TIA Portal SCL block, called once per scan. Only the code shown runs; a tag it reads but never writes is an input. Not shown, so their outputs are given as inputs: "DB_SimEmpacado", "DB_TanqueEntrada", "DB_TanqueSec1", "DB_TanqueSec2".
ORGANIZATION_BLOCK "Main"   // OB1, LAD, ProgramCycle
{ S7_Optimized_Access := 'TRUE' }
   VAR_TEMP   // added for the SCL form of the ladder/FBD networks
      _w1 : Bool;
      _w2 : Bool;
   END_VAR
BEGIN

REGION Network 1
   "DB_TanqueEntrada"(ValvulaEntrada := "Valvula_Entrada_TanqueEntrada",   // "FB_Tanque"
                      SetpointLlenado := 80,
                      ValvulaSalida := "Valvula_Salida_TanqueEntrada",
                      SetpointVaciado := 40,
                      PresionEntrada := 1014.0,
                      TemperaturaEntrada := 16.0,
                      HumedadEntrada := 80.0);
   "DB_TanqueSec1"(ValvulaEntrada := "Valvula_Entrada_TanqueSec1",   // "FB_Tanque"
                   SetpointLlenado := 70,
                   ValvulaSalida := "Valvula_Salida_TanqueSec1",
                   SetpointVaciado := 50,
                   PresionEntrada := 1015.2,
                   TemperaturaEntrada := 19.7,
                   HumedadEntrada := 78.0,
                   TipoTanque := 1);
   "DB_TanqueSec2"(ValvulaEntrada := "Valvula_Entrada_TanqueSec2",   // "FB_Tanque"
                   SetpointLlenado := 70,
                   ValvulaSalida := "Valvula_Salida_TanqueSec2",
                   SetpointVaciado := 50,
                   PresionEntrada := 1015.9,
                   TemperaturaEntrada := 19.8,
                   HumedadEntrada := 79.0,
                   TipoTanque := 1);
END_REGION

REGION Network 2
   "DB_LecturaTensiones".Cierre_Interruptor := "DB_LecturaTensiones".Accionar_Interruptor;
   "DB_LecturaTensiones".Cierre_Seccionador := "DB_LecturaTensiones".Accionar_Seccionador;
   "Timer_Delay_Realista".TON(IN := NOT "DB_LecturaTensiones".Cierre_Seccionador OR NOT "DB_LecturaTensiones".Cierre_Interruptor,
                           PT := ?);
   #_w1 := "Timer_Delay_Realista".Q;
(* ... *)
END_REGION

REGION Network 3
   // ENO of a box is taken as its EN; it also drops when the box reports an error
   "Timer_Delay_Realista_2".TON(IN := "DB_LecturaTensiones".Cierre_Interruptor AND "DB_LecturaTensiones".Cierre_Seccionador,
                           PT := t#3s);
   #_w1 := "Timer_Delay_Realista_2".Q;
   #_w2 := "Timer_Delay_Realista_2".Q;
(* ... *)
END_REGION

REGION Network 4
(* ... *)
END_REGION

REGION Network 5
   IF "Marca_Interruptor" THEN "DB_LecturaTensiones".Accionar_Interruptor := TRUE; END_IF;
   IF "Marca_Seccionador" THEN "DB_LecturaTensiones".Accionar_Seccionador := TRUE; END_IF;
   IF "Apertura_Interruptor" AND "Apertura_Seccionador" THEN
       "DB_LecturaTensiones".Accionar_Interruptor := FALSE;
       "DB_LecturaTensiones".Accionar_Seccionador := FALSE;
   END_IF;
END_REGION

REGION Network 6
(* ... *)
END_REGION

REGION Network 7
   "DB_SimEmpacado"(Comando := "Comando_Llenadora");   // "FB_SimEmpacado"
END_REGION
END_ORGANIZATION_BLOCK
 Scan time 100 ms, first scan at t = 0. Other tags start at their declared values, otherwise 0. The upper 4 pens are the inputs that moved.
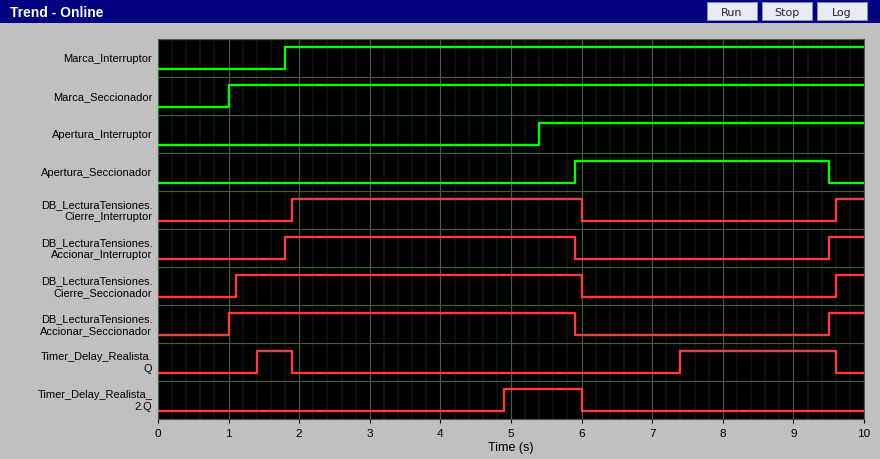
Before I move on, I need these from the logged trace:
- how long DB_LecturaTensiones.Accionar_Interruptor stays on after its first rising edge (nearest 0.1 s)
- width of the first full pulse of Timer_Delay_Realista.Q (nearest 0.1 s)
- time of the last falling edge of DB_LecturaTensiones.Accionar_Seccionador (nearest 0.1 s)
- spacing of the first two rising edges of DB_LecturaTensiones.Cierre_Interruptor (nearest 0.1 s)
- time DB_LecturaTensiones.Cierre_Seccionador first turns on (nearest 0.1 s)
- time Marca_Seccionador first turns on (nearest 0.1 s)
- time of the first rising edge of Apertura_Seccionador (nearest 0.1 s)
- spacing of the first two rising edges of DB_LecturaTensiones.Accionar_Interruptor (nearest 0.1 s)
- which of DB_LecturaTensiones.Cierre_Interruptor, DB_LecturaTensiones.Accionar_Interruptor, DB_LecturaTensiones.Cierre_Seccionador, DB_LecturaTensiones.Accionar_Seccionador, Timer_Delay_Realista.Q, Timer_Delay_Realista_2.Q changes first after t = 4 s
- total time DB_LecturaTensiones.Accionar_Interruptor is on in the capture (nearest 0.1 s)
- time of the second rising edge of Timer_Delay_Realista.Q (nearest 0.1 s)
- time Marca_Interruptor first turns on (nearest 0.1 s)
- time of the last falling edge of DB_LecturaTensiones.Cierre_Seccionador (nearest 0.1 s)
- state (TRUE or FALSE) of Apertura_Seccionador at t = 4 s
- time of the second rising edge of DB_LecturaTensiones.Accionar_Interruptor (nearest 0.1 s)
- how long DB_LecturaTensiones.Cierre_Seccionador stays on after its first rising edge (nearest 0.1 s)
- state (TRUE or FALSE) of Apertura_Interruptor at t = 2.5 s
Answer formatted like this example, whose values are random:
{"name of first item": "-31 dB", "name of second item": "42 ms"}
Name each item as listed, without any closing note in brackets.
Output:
{"how long DB_LecturaTensiones.Accionar_Interruptor stays on after its first rising edge": "4.1 s", "width of the first full pulse of Timer_Delay_Realista.Q": "0.5 s", "time of the last falling edge of DB_LecturaTensiones.Accionar_Seccionador": "5.9 s", "spacing of the first two rising edges of DB_LecturaTensiones.Cierre_Interruptor": "7.7 s", "time DB_LecturaTensiones.Cierre_Seccionador first turns on": "1.1 s", "time Marca_Seccionador first turns on": "1.0 s", "time of the first rising edge of Apertura_Seccionador": "5.9 s", "spacing of the first two rising edges of DB_LecturaTensiones.Accionar_Interruptor": "7.7 s", "which of DB_LecturaTensiones.Cierre_Interruptor, DB_LecturaTensiones.Accionar_Interruptor, DB_LecturaTensiones.Cierre_Seccionador, DB_LecturaTensiones.Accionar_Seccionador, Timer_Delay_Realista.Q, Timer_Delay_Realista_2.Q changes first after t = 4 s": "Timer_Delay_Realista_2.Q", "total time DB_LecturaTensiones.Accionar_Interruptor is on in the capture": "4.6 s", "time of the second rising edge of Timer_Delay_Realista.Q": "7.4 s", "time Marca_Interruptor first turns on": "1.8 s", "time of the last falling edge of DB_LecturaTensiones.Cierre_Seccionador": "6.0 s", "state (TRUE or FALSE) of Apertura_Seccionador at t = 4 s": "FALSE", "time of the second rising edge of DB_LecturaTensiones.Accionar_Interruptor": "9.5 s", "how long DB_LecturaTensiones.Cierre_Seccionador stays on after its first rising edge": "4.9 s", "state (TRUE or FALSE) of Apertura_Interruptor at t = 2.5 s": "FALSE"}
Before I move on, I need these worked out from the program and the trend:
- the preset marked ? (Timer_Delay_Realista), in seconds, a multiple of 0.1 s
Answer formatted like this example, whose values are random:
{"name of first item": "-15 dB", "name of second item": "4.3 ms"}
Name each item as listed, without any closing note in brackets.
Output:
{"the preset marked ? (Timer_Delay_Realista), in seconds, a multiple of 0.1 s": "1.4 s"}
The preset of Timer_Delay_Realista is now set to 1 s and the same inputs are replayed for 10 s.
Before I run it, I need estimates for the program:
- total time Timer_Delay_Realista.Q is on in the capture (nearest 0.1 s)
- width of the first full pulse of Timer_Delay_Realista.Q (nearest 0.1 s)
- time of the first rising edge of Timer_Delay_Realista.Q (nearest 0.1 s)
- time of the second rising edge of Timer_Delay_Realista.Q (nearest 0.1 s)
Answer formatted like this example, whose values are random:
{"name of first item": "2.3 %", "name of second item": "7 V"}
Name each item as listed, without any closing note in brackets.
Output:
{"total time Timer_Delay_Realista.Q is on in the capture": "3.5 s", "width of the first full pulse of Timer_Delay_Realista.Q": "0.9 s", "time of the first rising edge of Timer_Delay_Realista.Q": "1.0 s", "time of the second rising edge of Timer_Delay_Realista.Q": "7.0 s"}
